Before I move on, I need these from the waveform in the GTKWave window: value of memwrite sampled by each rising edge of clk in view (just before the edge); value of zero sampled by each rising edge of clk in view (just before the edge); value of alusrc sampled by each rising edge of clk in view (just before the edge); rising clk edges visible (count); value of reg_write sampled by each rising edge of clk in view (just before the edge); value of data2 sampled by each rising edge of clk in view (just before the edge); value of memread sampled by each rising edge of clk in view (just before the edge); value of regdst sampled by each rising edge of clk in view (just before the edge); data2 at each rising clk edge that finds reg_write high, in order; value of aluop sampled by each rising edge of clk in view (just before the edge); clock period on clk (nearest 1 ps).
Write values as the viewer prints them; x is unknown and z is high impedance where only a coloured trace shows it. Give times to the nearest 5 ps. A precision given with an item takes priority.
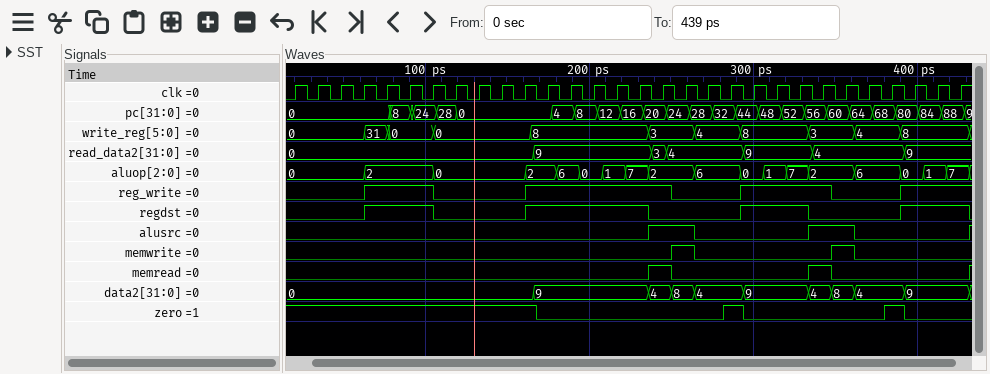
0 0 0 0 0 0 0 0 0 0 0 0 0 0 0 0 0 1 0 0 0 0 0 0 1 0 0 0 0 0
1 1 1 1 1 1 1 1 1 1 1 0 0 0 0 0 0 0 0 1 0 0 0 0 0 0 1 0 0 0
0 0 0 0 0 0 0 0 0 0 0 0 0 0 0 0 1 1 0 0 0 0 0 1 1 0 0 0 0 0
30
0 0 0 0 1 1 1 0 0 0 0 1 1 1 1 1 1 0 0 0 1 1 1 1 0 0 0 1 1 1
0, 0, 0, 0, 0, 0, 0, 0, 0, 0, 0, 9, 9, 9, 9, 9, 4, 8, 4, 4, 9, 9, 9, 4, 8, 4, 4, 9, 9, 9
0 0 0 0 0 0 0 0 0 0 0 0 0 0 0 0 1 0 0 0 0 0 0 1 0 0 0 0 0 0
0 0 0 0 1 1 1 0 0 0 0 1 1 1 1 1 0 0 0 0 1 1 1 0 0 0 0 1 1 1
0, 0, 0, 9, 9, 9, 9, 9, 4, 9, 9, 9, 4, 9, 9, 9
0, 0, 0, 0, 2, 2, 2, 0, 0, 0, 0, 2, 6, 0, 1, 7, 2, 2, 6, 6, 0, 1, 7, 2, 2, 6, 6, 0, 1, 7
14 ps
